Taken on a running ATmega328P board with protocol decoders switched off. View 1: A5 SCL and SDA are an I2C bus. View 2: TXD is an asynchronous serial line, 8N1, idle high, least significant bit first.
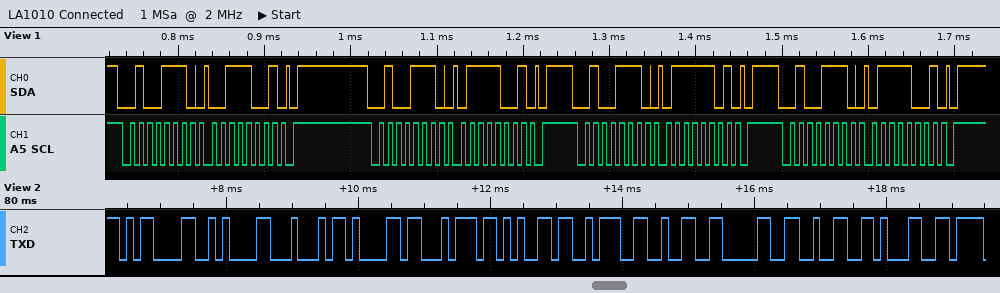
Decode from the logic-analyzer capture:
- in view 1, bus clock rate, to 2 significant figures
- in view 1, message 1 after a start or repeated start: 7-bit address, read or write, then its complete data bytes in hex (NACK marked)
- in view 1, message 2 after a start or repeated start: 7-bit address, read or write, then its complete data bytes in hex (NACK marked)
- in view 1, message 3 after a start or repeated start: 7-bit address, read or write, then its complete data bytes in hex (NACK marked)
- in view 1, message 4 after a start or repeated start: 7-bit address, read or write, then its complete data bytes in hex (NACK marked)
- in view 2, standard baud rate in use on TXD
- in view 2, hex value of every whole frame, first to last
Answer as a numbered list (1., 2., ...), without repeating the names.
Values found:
1. 100 kHz
2. 0x27 write: 39
3. 0x27 write: 79
4. 0x27 write: 7D
5. 0x27 write: 79
6. 9600 baud
7. 0x0D 0x0A 0x44 0x61 0x74 0x65 0x3A 0x32 0x30 0x32 0x31
